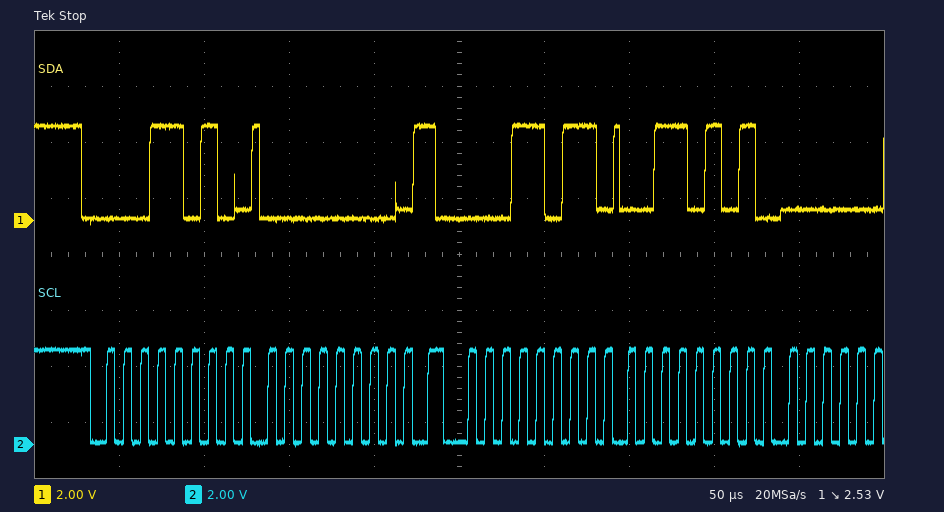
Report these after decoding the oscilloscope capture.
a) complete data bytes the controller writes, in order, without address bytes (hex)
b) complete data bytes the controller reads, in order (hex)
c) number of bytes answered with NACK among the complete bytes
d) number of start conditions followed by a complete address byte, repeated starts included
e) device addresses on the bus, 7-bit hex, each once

00
35
0
2
0x0D
